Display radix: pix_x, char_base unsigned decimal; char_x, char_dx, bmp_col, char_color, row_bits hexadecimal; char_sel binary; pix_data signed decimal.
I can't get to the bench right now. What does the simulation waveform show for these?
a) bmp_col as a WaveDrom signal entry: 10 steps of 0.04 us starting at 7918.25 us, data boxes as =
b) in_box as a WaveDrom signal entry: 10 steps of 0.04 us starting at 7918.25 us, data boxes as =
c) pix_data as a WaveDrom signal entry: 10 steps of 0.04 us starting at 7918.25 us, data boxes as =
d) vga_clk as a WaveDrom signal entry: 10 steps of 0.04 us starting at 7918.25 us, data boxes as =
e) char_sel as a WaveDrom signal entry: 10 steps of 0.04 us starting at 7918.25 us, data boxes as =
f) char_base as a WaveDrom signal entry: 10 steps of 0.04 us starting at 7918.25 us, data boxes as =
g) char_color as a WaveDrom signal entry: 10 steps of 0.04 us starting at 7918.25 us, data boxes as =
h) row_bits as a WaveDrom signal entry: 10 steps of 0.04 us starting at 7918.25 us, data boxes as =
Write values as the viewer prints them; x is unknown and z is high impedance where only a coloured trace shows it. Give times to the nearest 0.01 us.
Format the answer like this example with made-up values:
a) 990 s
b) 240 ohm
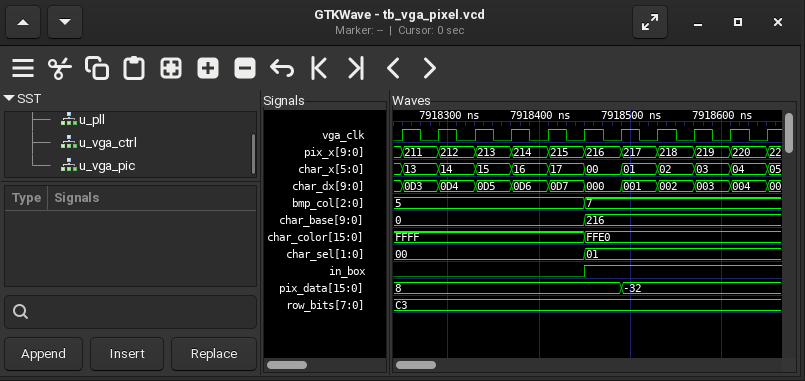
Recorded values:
a) {name: 'bmp_col', wave: '=....=....', data: '5 7'}
b) {name: 'in_box', wave: '0....1....'}
c) {name: 'pix_data', wave: '=.....=...', data: '8 -32'}
d) {name: 'vga_clk', wave: 'p.........'}
e) {name: 'char_sel', wave: '=....=....', data: '00 01'}
f) {name: 'char_base', wave: '=....=....', data: '0 216'}
g) {name: 'char_color', wave: '=....=....', data: 'FFFF FFE0'}
h) {name: 'row_bits', wave: '=.........', data: 'C3'}
